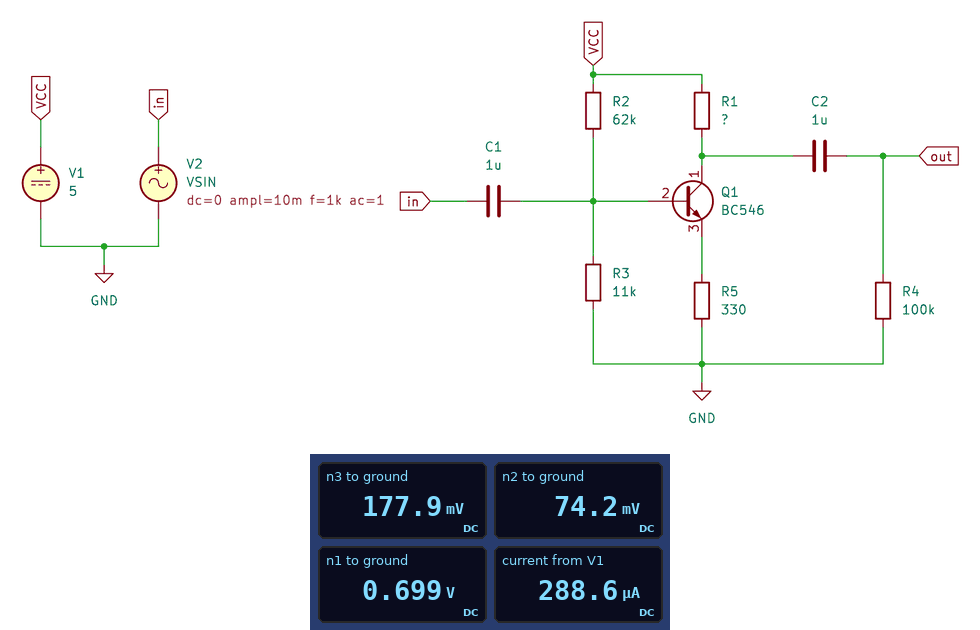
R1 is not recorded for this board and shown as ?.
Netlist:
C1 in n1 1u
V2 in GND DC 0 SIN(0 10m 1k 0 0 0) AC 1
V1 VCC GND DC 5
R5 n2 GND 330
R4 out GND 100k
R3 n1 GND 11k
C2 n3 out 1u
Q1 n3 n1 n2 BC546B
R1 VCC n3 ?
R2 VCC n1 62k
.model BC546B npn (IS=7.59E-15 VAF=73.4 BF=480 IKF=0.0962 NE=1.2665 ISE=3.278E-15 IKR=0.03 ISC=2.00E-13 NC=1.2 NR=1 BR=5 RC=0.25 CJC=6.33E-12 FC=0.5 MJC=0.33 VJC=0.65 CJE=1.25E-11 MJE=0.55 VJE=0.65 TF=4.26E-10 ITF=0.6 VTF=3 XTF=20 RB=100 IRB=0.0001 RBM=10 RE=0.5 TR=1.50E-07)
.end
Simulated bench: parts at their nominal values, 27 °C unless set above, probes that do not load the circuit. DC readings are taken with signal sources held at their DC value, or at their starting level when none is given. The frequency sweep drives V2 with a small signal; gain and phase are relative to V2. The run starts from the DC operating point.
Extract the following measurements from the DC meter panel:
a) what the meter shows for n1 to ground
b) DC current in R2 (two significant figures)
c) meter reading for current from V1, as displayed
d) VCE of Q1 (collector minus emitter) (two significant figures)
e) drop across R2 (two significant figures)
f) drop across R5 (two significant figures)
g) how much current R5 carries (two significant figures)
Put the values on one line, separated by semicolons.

0.699 V; 69 µA; 288.6 µA; 100 mV; 4.3 V; 74 mV; 220 µA
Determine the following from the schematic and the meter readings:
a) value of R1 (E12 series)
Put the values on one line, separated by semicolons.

22 kΩ
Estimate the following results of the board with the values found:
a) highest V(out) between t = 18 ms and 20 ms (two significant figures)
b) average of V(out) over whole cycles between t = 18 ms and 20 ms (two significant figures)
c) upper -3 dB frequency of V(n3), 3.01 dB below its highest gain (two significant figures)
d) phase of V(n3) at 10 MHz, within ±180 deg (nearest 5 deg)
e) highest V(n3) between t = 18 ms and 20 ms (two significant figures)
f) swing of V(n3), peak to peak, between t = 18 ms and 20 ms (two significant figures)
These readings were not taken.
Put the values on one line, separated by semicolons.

350 mV; 91 mV; 1.1 MHz; 45 deg; 550 mV; 400 mV
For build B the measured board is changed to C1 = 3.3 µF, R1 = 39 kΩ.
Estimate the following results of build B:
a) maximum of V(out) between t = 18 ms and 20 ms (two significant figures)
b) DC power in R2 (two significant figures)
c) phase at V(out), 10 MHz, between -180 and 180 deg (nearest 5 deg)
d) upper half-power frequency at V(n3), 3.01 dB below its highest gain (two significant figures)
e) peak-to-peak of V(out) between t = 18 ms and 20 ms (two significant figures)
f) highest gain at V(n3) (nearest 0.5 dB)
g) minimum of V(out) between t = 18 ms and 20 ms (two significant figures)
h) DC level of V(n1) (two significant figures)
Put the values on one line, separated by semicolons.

150 mV; 300 µW; 25 deg; 1.3 MHz; 170 mV; 9.0 dB; -20 mV; 660 mV
